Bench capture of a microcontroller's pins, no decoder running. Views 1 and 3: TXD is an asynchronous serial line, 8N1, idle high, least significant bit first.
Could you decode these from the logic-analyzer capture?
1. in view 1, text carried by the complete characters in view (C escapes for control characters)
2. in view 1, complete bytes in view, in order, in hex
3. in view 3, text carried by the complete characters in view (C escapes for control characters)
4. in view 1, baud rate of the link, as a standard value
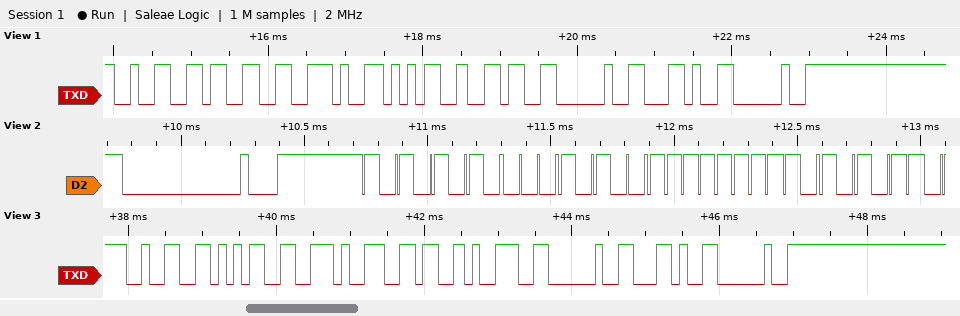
"23.56 , "
32 33 2E 35 36 20 2C 20
"25.69 , "
9600 baud
